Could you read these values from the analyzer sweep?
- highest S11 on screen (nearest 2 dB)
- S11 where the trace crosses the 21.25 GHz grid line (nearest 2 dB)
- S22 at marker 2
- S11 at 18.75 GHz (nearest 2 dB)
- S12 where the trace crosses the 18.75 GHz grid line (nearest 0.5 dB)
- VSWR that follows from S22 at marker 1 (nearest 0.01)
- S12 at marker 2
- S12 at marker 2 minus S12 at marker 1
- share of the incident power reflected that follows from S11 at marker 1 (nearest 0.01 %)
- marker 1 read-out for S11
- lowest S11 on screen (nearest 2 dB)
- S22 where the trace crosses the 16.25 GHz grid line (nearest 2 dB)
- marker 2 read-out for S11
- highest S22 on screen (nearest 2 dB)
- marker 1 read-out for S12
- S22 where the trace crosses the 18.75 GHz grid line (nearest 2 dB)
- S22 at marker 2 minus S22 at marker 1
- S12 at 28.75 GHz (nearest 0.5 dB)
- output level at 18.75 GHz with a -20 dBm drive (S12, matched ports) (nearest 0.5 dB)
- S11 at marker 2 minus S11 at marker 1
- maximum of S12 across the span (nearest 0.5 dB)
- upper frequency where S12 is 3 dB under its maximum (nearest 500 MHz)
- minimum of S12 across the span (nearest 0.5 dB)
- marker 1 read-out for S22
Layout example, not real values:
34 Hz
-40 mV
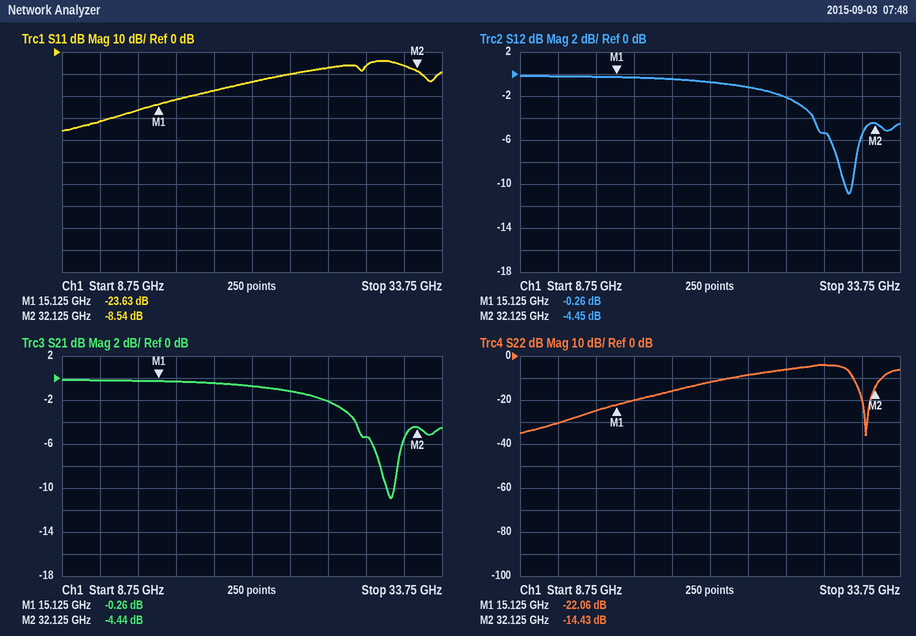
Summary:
-4 dB
-14 dB
-14.43 dB
-18 dB
-0.5 dB
1.17
-4.45 dB
-4.19 dB
0.43 %
-23.63 dB
-36 dB
-20 dB
-8.54 dB
-4 dB
-0.26 dB
-16 dB
7.63 dB
-5.5 dB
-20.5 dBm
15.09 dB
0.0 dB
27.5 GHz
-11.0 dB
-22.06 dB
